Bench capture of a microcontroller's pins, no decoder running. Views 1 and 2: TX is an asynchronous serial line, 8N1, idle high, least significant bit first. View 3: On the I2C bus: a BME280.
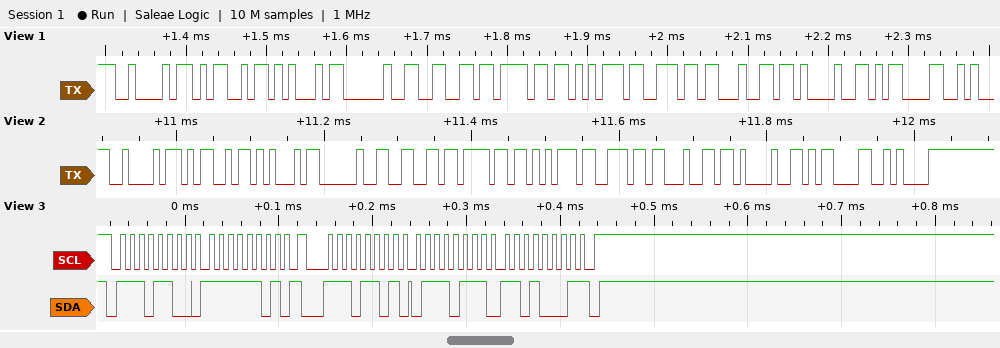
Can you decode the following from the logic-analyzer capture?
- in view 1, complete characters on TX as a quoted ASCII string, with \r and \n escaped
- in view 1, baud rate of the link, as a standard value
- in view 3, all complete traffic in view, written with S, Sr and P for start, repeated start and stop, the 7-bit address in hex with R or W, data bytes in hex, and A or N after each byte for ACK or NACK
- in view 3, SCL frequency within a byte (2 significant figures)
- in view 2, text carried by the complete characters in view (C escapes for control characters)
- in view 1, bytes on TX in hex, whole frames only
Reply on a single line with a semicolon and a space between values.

"BME found!\r"; 115200 baud; S 76W A FD A Sr 76R A 77 A D1 N P; 100 kHz; "BME found!\r\n"; 0x42 0x4D 0x45 0x20 0x66 0x6F 0x75 0x6E 0x64 0x21 0x0D
